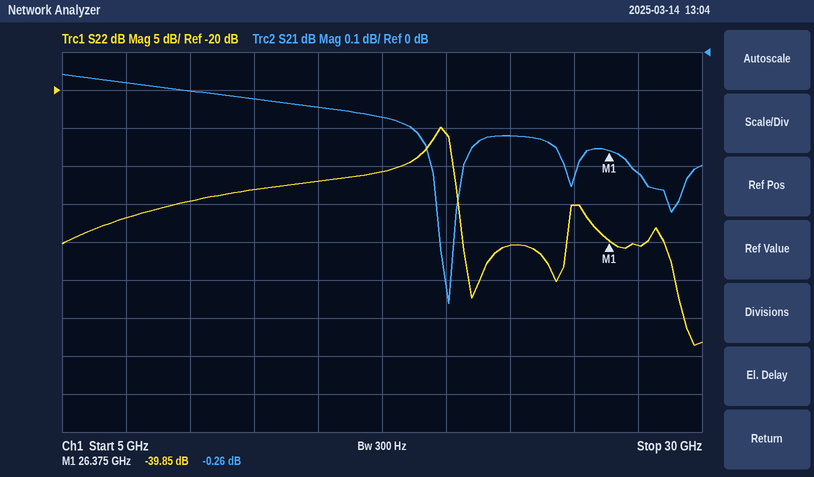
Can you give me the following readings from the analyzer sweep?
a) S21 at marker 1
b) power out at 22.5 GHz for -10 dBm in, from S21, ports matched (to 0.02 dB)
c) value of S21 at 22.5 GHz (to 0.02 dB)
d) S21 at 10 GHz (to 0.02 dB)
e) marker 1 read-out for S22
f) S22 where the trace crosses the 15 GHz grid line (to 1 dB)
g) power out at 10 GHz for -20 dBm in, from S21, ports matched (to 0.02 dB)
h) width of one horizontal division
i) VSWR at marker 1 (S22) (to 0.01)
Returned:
-0.26 dB
-10.22 dBm
-0.22 dB
-0.10 dB
-39.85 dB
-32 dB
-20.10 dBm
2.5 GHz
1.02
